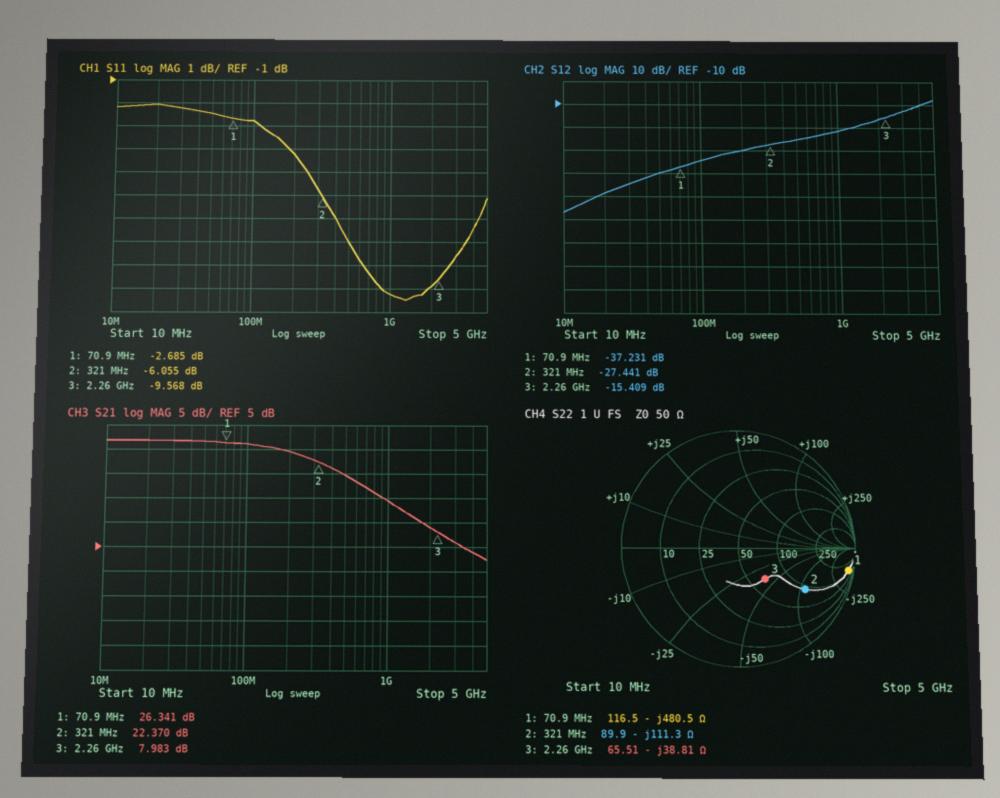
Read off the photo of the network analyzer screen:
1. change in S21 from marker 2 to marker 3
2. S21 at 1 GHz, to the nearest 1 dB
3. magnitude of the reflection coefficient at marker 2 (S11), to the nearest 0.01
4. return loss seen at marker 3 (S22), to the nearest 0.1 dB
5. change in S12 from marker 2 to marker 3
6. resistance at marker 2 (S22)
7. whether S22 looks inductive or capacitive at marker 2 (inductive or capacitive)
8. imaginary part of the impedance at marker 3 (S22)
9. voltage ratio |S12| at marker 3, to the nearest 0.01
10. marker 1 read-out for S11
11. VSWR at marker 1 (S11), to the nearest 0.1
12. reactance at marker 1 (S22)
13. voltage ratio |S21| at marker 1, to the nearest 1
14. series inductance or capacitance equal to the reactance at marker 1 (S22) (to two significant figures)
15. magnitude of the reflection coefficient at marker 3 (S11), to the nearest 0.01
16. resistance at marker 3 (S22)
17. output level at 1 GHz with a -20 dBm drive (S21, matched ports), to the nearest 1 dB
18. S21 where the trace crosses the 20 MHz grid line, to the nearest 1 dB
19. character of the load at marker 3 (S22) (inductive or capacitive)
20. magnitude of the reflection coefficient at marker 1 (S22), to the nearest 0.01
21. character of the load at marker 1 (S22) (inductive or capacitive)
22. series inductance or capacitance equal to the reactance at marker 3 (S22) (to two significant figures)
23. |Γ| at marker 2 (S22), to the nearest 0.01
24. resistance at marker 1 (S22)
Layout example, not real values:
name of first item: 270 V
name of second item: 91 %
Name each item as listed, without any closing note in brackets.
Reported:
change in S21 from marker 2 to marker 3: -14.387 dB
S21 at 1 GHz, to the nearest 1 dB: 14 dB
magnitude of the reflection coefficient at marker 2 (S11), to the nearest 0.01: 0.50
return loss seen at marker 3 (S22), to the nearest 0.1 dB: 9.3 dB
change in S12 from marker 2 to marker 3: 12.032 dB
resistance at marker 2: 89.9 Ω
whether S22 looks inductive or capacitive at marker 2: capacitive
imaginary part of the impedance at marker 3: -38.81 Ω
voltage ratio |S12| at marker 3, to the nearest 0.01: 0.17
marker 1 read-out for S11: -2.685 dB
VSWR at marker 1 (S11), to the nearest 0.1: 6.5
reactance at marker 1: -480.5 Ω
voltage ratio |S21| at marker 1, to the nearest 1: 21
series inductance or capacitance equal to the reactance at marker 1 (S22): 4.7 pF
magnitude of the reflection coefficient at marker 3 (S11), to the nearest 0.01: 0.33
resistance at marker 3: 65.51 Ω
output level at 1 GHz with a -20 dBm drive (S21, matched ports), to the nearest 1 dB: -6 dBm
S21 where the trace crosses the 20 MHz grid line, to the nearest 1 dB: 27 dB
character of the load at marker 3 (S22): capacitive
magnitude of the reflection coefficient at marker 1 (S22), to the nearest 0.01: 0.95
character of the load at marker 1 (S22): capacitive
series inductance or capacitance equal to the reactance at marker 3 (S22): 1.8 pF
|Γ| at marker 2 (S22), to the nearest 0.01: 0.66
resistance at marker 1: 116.5 Ω
